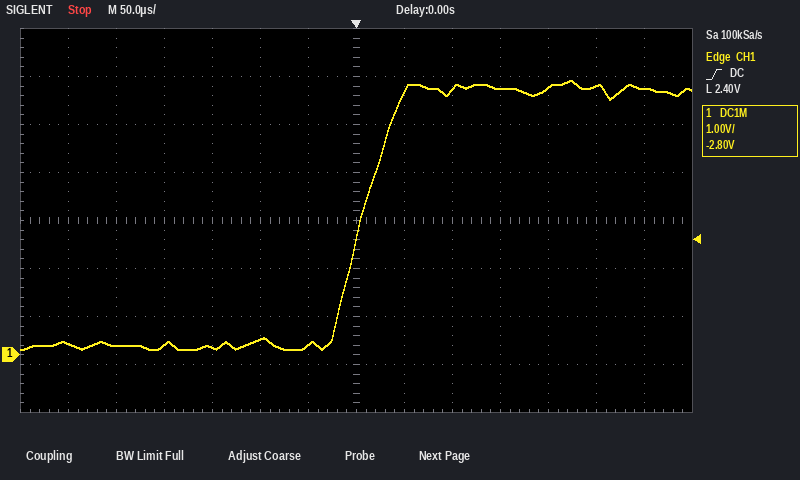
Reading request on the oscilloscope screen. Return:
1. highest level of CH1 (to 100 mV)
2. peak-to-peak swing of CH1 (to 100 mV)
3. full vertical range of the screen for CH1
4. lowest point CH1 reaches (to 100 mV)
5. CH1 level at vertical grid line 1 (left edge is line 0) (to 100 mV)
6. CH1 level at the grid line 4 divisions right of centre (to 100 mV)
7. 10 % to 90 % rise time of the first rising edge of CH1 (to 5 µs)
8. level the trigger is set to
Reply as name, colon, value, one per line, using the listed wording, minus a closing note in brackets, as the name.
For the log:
highest level of CH1: 5.7 V
peak-to-peak swing of CH1: 5.6 V
full vertical range of the screen for CH1: 8 V
lowest point CH1 reaches: 100 mV
CH1 level at vertical grid line 1 (left edge is line 0): 200 mV
CH1 level at the grid line 4 divisions right of centre: 5.6 V
10 % to 90 % rise time of the first rising edge of CH1: 60 µs
level the trigger is set to: 2.40 V
